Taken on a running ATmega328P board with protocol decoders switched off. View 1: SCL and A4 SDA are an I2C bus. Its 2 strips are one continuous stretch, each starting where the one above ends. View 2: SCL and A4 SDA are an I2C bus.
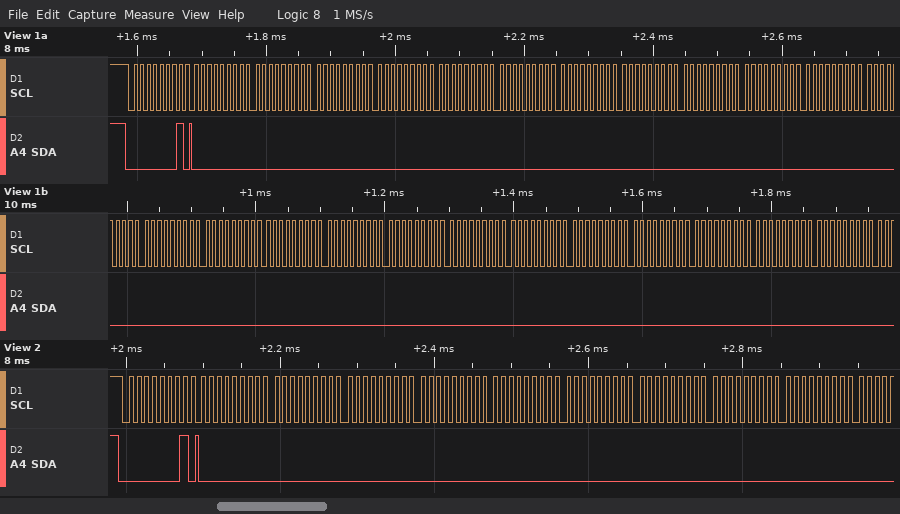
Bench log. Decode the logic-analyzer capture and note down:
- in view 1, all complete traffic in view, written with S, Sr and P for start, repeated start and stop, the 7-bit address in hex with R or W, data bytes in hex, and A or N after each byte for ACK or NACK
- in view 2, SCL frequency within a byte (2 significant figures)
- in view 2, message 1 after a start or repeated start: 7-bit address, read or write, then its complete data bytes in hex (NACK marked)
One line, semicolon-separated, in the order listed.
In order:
S 00R A 00 A 00 A 00 A 00 A 00 A 00 A 00 A 00 A 00 A 00 A 00 A 00 A 00 A 00 A 00 A 00 A 00 A 00 A 00 A 00 A 00 A 00 A 00 A 00 A; 100 kHz; 0x00 read: 00 00 00 00 00 00 00 00 00
